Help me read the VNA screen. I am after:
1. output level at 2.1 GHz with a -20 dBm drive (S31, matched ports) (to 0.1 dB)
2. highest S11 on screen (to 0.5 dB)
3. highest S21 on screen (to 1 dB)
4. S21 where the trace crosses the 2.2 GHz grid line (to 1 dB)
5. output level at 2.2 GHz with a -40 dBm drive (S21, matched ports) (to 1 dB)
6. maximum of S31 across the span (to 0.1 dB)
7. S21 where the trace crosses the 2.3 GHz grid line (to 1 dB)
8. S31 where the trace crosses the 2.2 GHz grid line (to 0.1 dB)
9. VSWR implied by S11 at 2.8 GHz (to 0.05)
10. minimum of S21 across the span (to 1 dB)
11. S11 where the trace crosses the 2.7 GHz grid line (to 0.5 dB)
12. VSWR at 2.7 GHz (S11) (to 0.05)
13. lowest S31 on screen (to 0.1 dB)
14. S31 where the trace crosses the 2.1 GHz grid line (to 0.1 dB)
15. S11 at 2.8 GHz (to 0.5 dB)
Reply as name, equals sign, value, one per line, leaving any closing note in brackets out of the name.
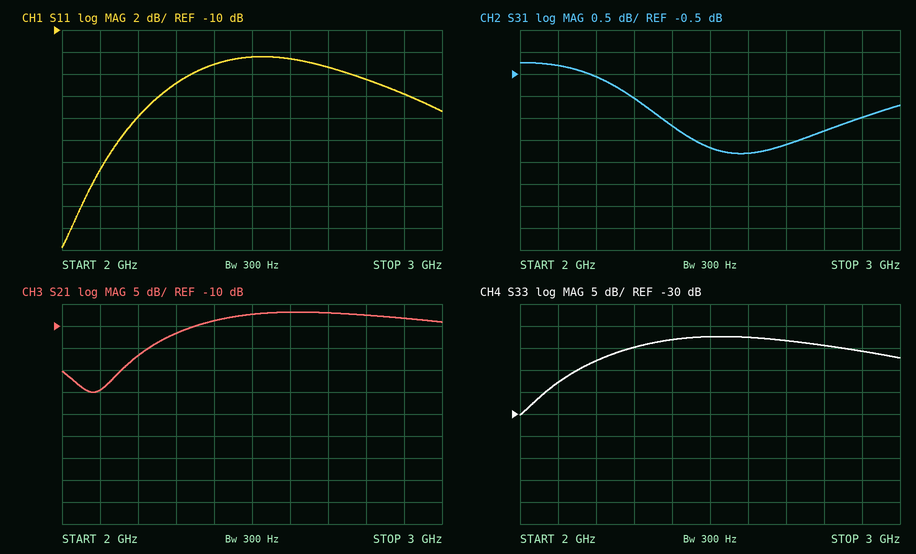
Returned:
output level at 2.1 GHz with a -20 dBm drive (S31, matched ports) = -20.3 dBm
highest S11 on screen = -12.5 dB
highest S21 on screen = -7 dB
S21 where the trace crosses the 2.2 GHz grid line = -17 dB
output level at 2.2 GHz with a -40 dBm drive (S21, matched ports) = -57 dBm
maximum of S31 across the span = -0.2 dB
S21 where the trace crosses the 2.3 GHz grid line = -12 dB
S31 where the trace crosses the 2.2 GHz grid line = -0.6 dB
VSWR implied by S11 at 2.8 GHz = 1.45
minimum of S21 across the span = -25 dB
S11 where the trace crosses the 2.7 GHz grid line = -13.5 dB
VSWR at 2.7 GHz (S11) = 1.55
lowest S31 on screen = -2.3 dB
S31 where the trace crosses the 2.1 GHz grid line = -0.3 dB
S11 at 2.8 GHz = -14.5 dB
